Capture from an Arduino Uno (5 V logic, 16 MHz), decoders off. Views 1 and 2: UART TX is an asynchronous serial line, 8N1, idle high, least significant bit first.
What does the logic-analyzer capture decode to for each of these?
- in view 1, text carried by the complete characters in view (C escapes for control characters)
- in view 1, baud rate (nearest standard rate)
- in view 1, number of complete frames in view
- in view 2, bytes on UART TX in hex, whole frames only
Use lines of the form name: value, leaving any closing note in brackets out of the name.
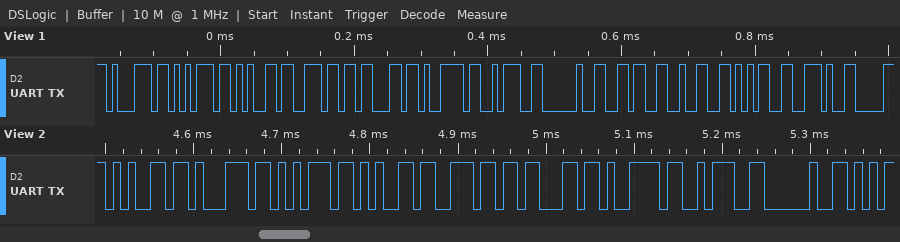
in view 1, text carried by the complete characters in view: "quency: 625."
in view 1, baud rate: 115200 baud
in view 1, number of complete frames in view: 12
in view 2, bytes on UART TX in hex, whole frames only: 65 71 75 65 6E 63 79 3A 20
